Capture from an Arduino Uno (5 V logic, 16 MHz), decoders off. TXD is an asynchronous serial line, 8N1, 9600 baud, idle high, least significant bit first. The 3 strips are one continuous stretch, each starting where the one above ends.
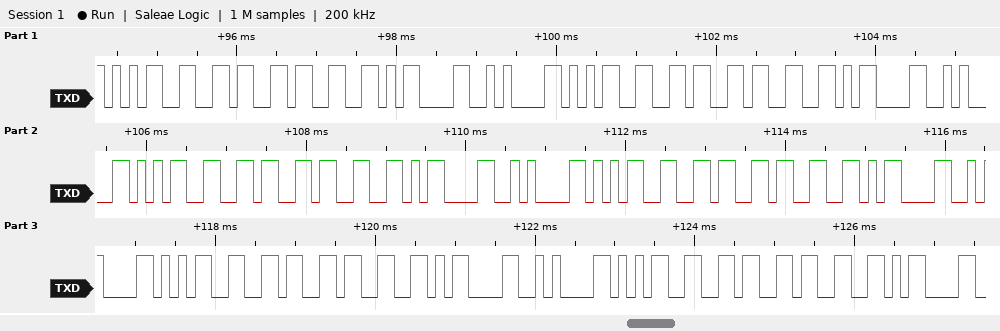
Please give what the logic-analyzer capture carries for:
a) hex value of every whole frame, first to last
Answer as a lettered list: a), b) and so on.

a) 35 36 33 0D 0A 35 36 33 0D 0A 35 36 33 0D 0A 35 36 33 0D 0A 35 36 33 0D 0A 35 36 33 0D
